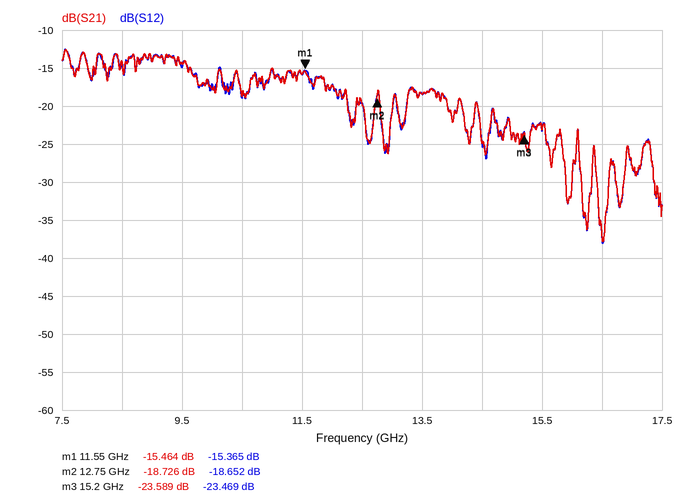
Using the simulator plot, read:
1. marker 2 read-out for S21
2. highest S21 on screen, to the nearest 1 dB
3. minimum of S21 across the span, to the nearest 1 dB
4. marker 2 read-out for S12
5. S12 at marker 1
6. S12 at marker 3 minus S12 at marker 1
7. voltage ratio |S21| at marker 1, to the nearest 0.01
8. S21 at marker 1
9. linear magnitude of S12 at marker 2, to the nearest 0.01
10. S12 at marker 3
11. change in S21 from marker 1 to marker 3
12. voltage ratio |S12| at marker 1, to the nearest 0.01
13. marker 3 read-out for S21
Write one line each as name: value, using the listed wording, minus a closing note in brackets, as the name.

marker 2 read-out for S21: -18.726 dB
highest S21 on screen, to the nearest 1 dB: -13 dB
minimum of S21 across the span, to the nearest 1 dB: -38 dB
marker 2 read-out for S12: -18.652 dB
S12 at marker 1: -15.365 dB
S12 at marker 3 minus S12 at marker 1: -8.104 dB
voltage ratio |S21| at marker 1, to the nearest 0.01: 0.17
S21 at marker 1: -15.464 dB
linear magnitude of S12 at marker 2, to the nearest 0.01: 0.12
S12 at marker 3: -23.469 dB
change in S21 from marker 1 to marker 3: -8.125 dB
voltage ratio |S12| at marker 1, to the nearest 0.01: 0.17
marker 3 read-out for S21: -23.589 dB
